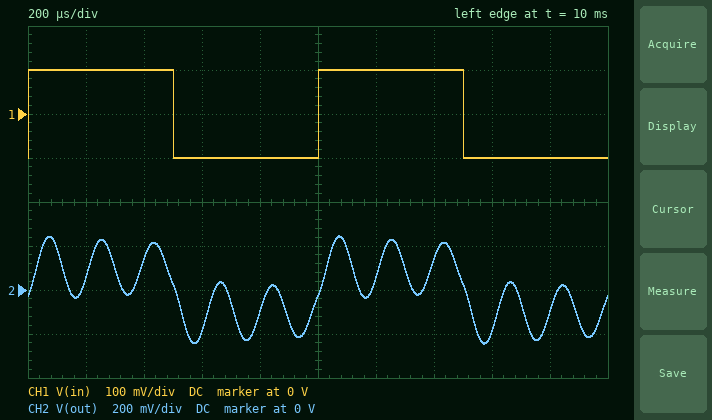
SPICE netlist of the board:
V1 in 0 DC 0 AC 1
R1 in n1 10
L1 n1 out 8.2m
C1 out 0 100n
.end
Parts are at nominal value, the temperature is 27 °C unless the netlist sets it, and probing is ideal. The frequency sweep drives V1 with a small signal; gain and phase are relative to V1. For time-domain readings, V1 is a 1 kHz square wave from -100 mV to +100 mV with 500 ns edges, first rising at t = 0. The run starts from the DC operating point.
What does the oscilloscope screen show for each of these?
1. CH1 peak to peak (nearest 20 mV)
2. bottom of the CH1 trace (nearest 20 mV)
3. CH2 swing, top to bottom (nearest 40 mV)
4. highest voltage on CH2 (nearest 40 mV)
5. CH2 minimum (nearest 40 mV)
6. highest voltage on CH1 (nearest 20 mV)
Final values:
200 mV
-100 mV
480 mV
240 mV
-240 mV
100 mV
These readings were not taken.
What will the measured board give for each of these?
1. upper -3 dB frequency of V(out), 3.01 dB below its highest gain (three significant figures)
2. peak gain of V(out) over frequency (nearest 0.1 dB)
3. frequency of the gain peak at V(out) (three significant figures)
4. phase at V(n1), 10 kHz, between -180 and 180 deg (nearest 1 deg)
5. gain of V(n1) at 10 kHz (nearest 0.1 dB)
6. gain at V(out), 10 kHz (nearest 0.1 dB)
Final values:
5.65 kHz
29.1 dB
5.56 kHz
2 deg
0 dB
-7.0 dB
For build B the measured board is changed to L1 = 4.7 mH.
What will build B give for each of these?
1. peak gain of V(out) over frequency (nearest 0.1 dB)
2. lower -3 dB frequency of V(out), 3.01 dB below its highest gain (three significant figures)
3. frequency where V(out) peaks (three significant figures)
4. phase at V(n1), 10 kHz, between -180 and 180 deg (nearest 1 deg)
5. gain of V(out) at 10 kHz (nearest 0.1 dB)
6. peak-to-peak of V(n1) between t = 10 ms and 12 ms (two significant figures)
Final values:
26.7 dB
7.17 kHz
7.34 kHz
4 deg
1.3 dB
220 mV
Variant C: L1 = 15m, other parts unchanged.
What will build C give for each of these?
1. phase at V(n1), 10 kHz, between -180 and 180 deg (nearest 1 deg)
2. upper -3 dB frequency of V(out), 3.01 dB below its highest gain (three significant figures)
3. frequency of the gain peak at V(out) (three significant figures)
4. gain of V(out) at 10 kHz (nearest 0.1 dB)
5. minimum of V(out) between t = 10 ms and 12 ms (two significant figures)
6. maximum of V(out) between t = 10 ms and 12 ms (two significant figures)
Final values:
1 deg
4.16 kHz
4.11 kHz
-13.8 dB
-210 mV
210 mV
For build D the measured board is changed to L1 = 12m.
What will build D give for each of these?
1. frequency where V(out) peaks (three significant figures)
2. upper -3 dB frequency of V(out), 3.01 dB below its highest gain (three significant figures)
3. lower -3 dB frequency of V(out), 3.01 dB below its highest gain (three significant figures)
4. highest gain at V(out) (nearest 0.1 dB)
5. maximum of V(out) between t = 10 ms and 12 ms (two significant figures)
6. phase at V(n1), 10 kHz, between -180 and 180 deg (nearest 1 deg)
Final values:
4.59 kHz
4.66 kHz
4.53 kHz
30.8 dB
270 mV
1 deg
